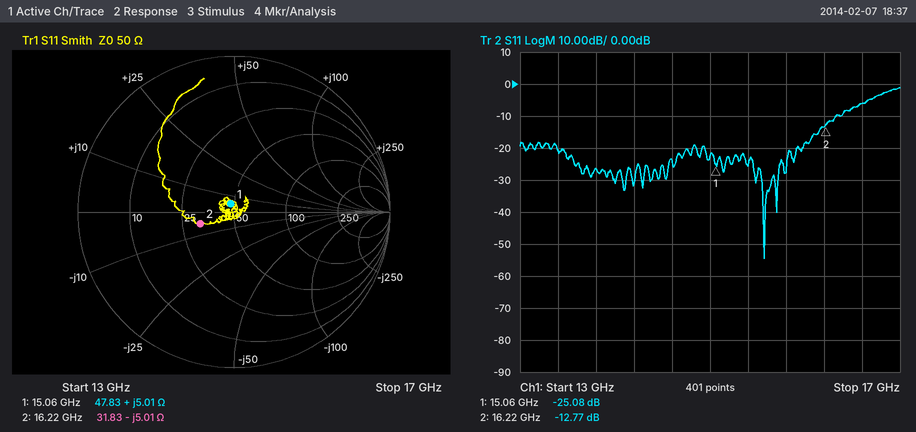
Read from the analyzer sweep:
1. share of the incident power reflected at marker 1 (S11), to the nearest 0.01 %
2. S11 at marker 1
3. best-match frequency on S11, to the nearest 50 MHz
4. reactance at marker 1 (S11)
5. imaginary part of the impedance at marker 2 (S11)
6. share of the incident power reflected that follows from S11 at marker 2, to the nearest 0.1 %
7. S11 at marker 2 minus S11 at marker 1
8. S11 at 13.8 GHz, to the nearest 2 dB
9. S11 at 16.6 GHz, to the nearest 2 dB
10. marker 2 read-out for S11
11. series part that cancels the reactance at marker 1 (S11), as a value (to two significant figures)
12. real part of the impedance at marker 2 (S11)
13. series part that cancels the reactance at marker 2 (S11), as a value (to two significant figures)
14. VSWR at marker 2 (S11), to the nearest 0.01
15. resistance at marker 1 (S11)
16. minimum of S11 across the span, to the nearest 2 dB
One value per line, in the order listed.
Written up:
0.31 %
-25.08 dB
15.55 GHz
+5.01 Ω
-5.01 Ω
5.3 %
12.31 dB
-26 dB
-6 dB
-12.77 dB
2.1 pF
31.83 Ω
49 pH
1.60
47.83 Ω
-54 dB
